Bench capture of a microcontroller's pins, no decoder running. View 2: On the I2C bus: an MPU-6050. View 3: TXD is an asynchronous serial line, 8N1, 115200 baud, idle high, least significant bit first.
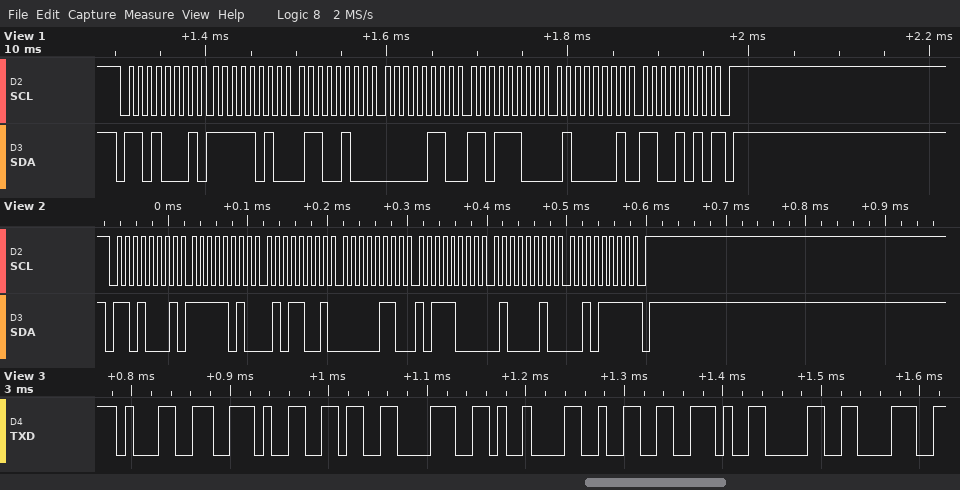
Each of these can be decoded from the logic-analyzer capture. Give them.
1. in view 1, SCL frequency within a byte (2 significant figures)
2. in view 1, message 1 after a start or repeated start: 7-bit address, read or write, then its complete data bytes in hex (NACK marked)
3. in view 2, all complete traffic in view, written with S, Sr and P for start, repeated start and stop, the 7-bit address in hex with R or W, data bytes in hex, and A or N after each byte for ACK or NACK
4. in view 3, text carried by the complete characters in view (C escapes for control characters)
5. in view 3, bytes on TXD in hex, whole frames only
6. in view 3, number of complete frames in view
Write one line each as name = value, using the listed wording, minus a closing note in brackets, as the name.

in view 1, SCL frequency within a byte = 100 kHz
in view 1, message 1 after a start or repeated start: 7-bit address, read or write, then its complete data bytes in hex = 0x68 read: FA 64 06 DC 41 CA NACK
in view 2, all complete traffic in view, written with S, Sr and P for start, repeated start and stop, the 7-bit address in hex with R or W, data bytes in hex, and A or N after each byte for ACK or NACK = S 68R A FA A 59 A 06 A B8 A 42 A 2F N P
in view 3, text carried by the complete characters in view = "1.68\t2.08"
in view 3, bytes on TXD in hex, whole frames only = 31 2E 36 38 09 32 2E 30 38
in view 3, number of complete frames in view = 9
